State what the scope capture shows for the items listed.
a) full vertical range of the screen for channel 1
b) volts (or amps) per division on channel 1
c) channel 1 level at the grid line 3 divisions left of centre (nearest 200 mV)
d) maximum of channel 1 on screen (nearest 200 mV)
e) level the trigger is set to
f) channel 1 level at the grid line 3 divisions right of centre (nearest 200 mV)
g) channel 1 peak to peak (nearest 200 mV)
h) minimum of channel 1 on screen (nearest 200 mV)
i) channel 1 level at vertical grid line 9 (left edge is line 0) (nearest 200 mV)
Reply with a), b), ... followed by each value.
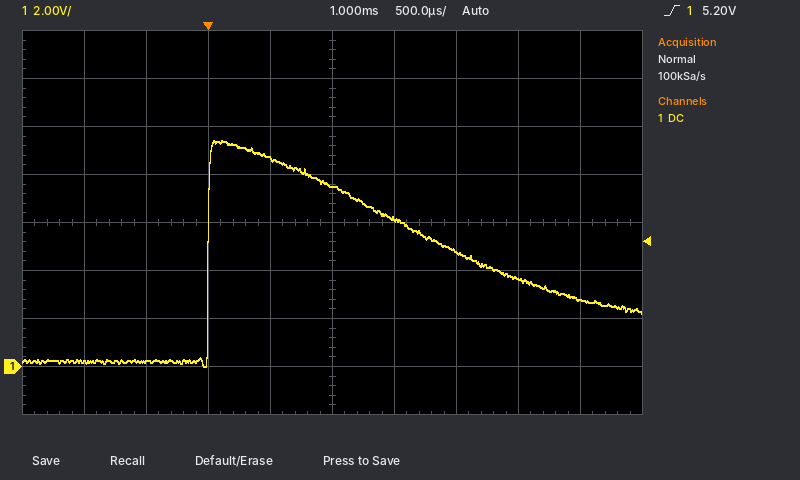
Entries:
a) 16 V
b) 2 V
c) 200 mV
d) 9.4 V
e) 5.20 V
f) 3.6 V
g) 9.4 V
h) 0.0 V
i) 2.8 V
